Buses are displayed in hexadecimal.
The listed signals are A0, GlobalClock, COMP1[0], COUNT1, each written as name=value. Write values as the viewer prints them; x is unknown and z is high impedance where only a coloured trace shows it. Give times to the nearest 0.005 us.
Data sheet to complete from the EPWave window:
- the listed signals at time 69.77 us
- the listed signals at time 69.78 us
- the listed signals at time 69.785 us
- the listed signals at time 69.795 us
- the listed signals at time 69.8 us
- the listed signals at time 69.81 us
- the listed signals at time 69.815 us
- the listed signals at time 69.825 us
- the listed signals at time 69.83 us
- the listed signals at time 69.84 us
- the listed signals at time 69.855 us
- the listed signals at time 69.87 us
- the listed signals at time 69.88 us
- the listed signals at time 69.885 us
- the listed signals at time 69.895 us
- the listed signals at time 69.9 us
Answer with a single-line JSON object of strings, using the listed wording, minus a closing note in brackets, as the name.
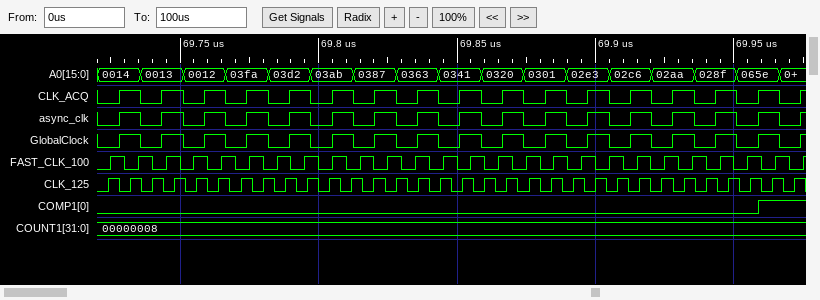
{"the listed signals at time 69.77 us": "A0=03fa, GlobalClock=0, COMP1[0]=0, COUNT1=00000008", "the listed signals at time 69.78 us": "A0=03fa, GlobalClock=1, COMP1[0]=0, COUNT1=00000008", "the listed signals at time 69.785 us": "A0=03d2, GlobalClock=0, COMP1[0]=0, COUNT1=00000008", "the listed signals at time 69.795 us": "A0=03d2, GlobalClock=1, COMP1[0]=0, COUNT1=00000008", "the listed signals at time 69.8 us": "A0=03ab, GlobalClock=0, COMP1[0]=0, COUNT1=00000008", "the listed signals at time 69.81 us": "A0=03ab, GlobalClock=1, COMP1[0]=0, COUNT1=00000008", "the listed signals at time 69.815 us": "A0=0387, GlobalClock=0, COMP1[0]=0, COUNT1=00000008", "the listed signals at time 69.825 us": "A0=0387, GlobalClock=1, COMP1[0]=0, COUNT1=00000008", "the listed signals at time 69.83 us": "A0=0363, GlobalClock=0, COMP1[0]=0, COUNT1=00000008", "the listed signals at time 69.84 us": "A0=0363, GlobalClock=1, COMP1[0]=0, COUNT1=00000008", "the listed signals at time 69.855 us": "A0=0341, GlobalClock=1, COMP1[0]=0, COUNT1=00000008", "the listed signals at time 69.87 us": "A0=0320, GlobalClock=1, COMP1[0]=0, COUNT1=00000008", "the listed signals at time 69.88 us": "A0=0301, GlobalClock=0, COMP1[0]=0, COUNT1=00000008", "the listed signals at time 69.885 us": "A0=0301, GlobalClock=1, COMP1[0]=0, COUNT1=00000008", "the listed signals at time 69.895 us": "A0=02e3, GlobalClock=0, COMP1[0]=0, COUNT1=00000008", "the listed signals at time 69.9 us": "A0=02e3, GlobalClock=1, COMP1[0]=0, COUNT1=00000008"}
